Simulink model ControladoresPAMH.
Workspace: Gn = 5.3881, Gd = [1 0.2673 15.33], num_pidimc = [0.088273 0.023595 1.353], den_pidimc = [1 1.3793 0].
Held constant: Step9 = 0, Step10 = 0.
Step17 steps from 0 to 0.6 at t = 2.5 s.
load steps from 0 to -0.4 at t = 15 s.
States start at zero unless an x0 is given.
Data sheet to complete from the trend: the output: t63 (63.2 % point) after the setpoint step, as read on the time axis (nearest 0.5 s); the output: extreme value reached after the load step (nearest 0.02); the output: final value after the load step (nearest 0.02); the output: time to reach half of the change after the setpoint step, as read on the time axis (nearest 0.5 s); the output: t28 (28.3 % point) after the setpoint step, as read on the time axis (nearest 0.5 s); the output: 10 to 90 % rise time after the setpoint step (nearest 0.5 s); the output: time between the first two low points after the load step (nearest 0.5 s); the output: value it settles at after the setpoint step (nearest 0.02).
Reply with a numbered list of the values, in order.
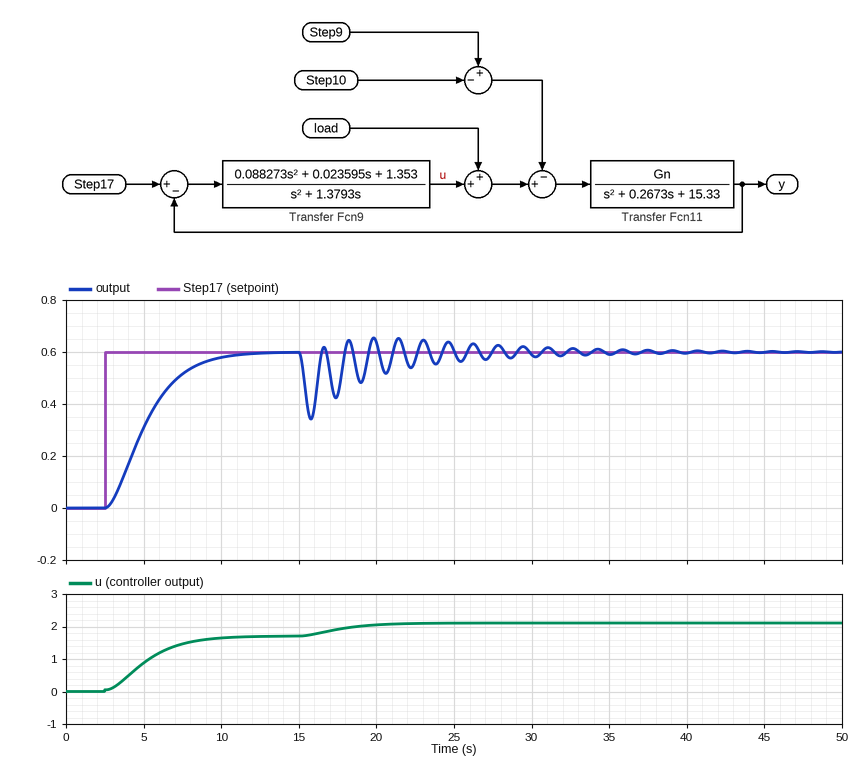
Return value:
1. 5.5 s
2. 0.34
3. 0.60
4. 5.0 s
5. 4.0 s
6. 5.0 s
7. 1.5 s
8. 0.60
